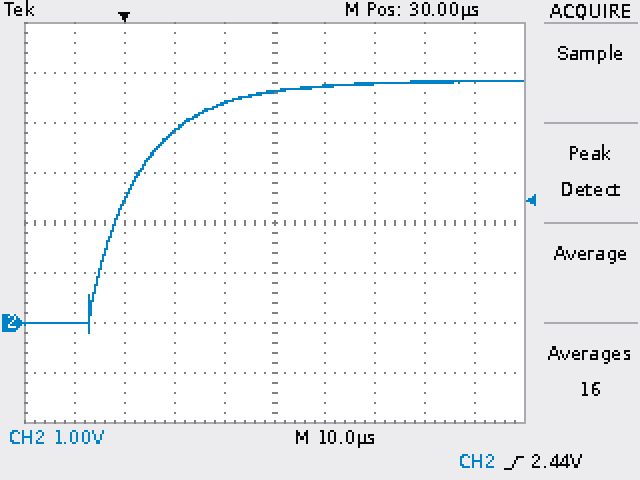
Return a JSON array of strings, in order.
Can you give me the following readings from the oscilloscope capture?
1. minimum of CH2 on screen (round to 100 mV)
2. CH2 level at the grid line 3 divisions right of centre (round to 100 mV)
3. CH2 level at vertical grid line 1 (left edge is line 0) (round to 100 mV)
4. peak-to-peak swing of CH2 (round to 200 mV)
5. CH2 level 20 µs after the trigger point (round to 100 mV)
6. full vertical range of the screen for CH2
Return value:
["-200 mV", "4.8 V", "0.0 V", "5.0 V", "4.4 V", "8 V"]
